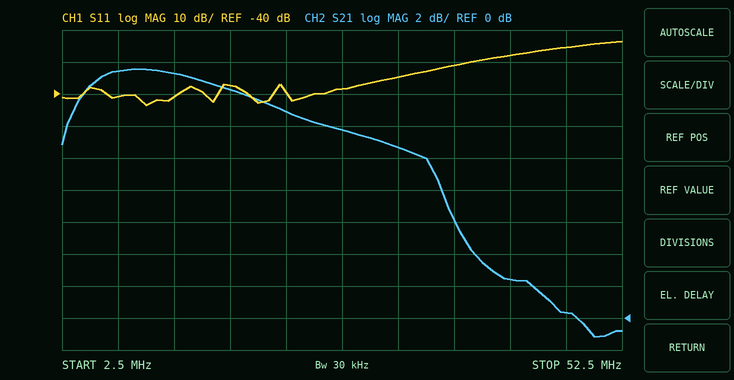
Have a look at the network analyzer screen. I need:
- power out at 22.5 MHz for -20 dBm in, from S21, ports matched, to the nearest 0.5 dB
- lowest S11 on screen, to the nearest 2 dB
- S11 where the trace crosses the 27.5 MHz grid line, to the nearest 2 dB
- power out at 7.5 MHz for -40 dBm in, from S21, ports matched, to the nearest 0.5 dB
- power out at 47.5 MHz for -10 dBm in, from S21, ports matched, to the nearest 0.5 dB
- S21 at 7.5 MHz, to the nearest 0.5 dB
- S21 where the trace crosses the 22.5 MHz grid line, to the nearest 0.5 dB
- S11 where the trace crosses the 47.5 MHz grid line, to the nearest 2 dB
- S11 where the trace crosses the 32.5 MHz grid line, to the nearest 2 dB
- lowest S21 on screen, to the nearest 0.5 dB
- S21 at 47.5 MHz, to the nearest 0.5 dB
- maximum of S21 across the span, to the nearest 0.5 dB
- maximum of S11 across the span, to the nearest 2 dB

-7.0 dBm
-44 dB
-38 dB
-24.5 dBm
-9.5 dBm
15.5 dB
13.0 dB
-26 dB
-34 dB
-1.0 dB
0.5 dB
15.5 dB
-24 dB
